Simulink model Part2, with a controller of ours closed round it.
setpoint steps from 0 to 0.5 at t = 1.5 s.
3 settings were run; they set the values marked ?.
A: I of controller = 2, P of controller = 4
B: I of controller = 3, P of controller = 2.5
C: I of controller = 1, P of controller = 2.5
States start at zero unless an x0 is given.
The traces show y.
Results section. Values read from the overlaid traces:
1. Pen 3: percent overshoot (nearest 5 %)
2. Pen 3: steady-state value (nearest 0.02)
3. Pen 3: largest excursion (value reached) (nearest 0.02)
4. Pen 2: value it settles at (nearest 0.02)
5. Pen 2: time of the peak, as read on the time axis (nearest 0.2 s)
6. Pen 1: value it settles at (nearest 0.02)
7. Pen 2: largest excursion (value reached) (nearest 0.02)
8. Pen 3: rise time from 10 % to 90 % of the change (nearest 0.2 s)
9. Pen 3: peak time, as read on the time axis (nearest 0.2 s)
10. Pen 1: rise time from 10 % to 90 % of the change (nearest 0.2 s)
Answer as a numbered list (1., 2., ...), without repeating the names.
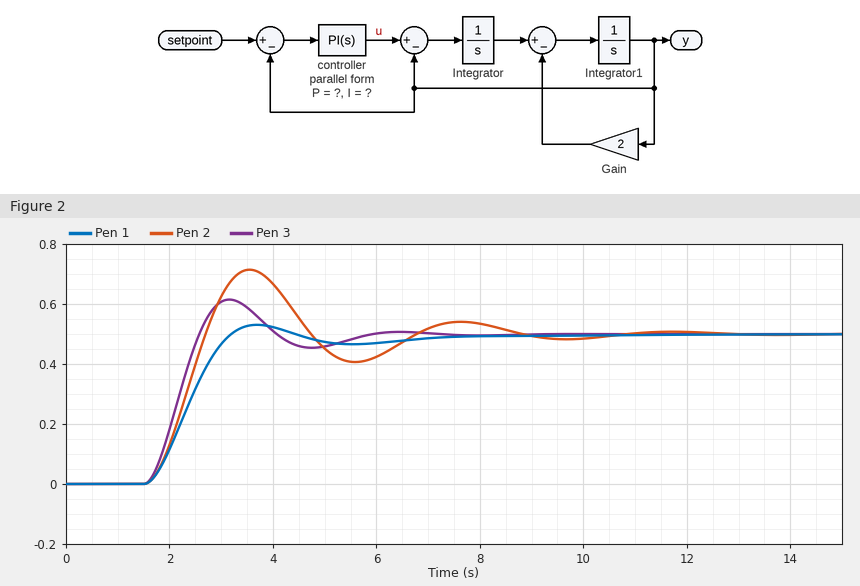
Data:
1. 25 %
2. 0.50
3. 0.62
4. 0.50
5. 3.6 s
6. 0.50
7. 0.72
8. 0.8 s
9. 3.2 s
10. 1.2 s
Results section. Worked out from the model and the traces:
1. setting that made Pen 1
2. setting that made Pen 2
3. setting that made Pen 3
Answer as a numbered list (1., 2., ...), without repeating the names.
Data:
1. C
2. B
3. A
